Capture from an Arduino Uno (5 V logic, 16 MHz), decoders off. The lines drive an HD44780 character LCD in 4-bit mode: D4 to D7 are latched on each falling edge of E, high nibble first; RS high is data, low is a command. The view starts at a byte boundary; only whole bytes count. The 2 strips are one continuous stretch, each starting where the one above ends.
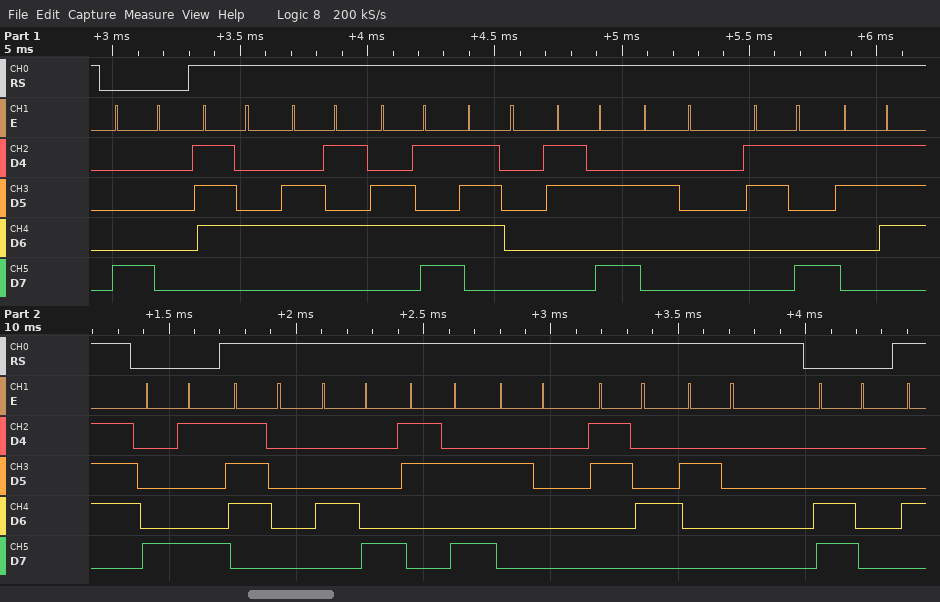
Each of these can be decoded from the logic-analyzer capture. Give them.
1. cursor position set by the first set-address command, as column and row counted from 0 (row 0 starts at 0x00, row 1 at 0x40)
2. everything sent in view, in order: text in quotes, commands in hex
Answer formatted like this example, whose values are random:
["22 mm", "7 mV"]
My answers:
["column 0, row 0", "0x80 \"temp: 97\" 0x89 \"pH: 4 \" 0xC0"]
